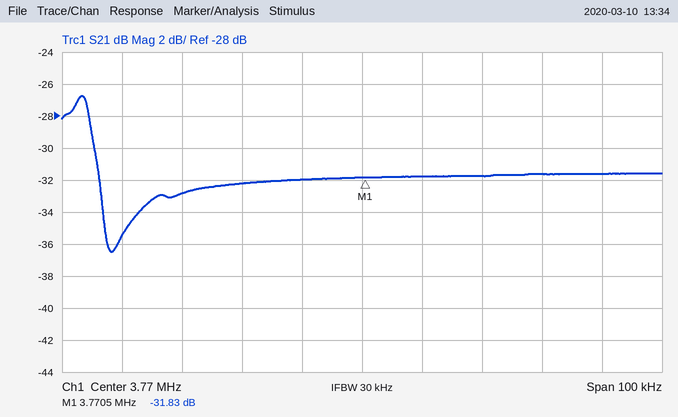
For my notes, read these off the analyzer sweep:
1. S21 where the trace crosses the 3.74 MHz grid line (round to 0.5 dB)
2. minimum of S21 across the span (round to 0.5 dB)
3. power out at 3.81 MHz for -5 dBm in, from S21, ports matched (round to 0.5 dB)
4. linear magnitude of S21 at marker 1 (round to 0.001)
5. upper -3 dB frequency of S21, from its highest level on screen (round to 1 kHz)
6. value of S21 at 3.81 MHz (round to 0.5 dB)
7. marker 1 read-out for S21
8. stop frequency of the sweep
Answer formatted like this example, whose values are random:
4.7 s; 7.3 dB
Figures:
-33.0 dB; -36.5 dB; -36.5 dBm; 0.026; 3.725 MHz; -31.5 dB; -31.83 dB; 3.82 MHz
